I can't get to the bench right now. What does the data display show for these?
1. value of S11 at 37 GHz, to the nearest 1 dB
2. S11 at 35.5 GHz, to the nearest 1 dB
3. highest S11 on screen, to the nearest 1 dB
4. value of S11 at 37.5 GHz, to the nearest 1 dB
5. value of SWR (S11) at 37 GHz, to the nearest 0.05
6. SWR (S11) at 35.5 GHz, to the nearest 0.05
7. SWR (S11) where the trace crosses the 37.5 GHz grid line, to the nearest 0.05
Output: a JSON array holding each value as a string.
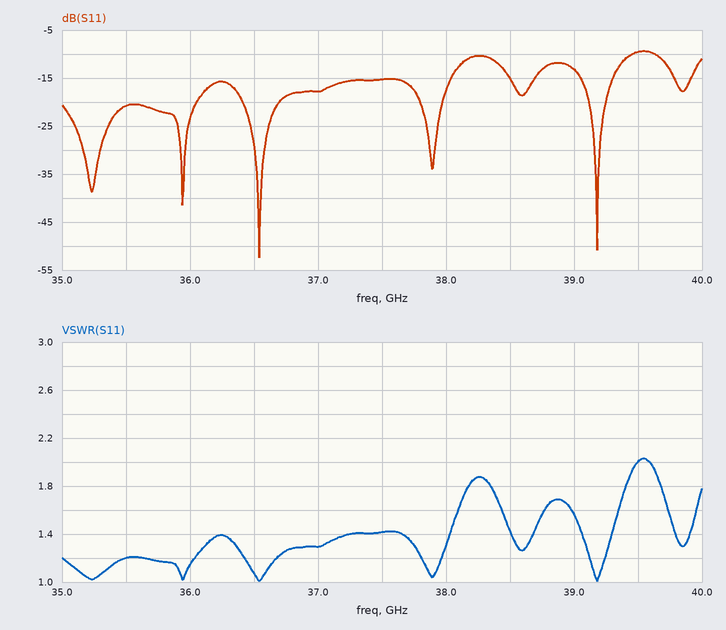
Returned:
["-18 dB", "-21 dB", "-9 dB", "-15 dB", "1.30", "1.20", "1.40"]
